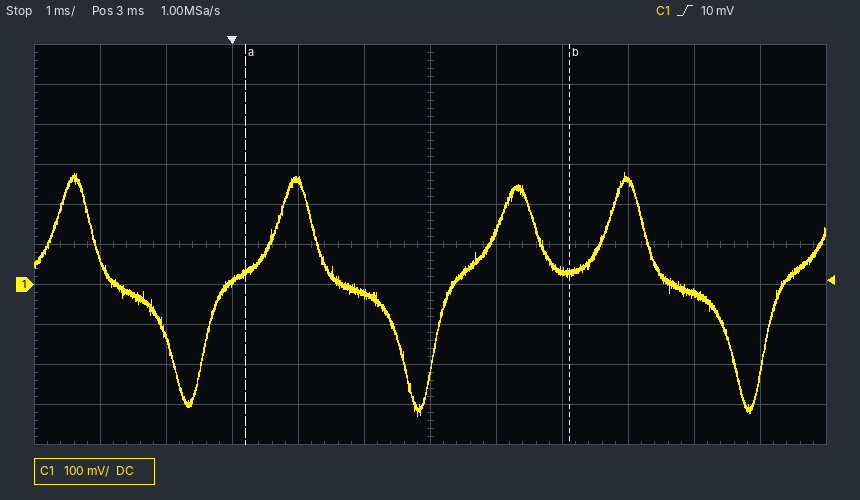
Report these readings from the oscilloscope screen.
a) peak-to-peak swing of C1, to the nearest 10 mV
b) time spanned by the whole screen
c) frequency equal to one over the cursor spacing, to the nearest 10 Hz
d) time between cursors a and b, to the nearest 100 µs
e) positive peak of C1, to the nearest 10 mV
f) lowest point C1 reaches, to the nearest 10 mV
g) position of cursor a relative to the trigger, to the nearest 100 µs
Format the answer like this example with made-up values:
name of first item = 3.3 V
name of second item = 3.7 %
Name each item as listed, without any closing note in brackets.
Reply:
peak-to-peak swing of C1, to the nearest 10 mV = 610 mV
time spanned by the whole screen = 12 ms
frequency equal to one over the cursor spacing, to the nearest 10 Hz = 200 Hz
time between cursors a and b, to the nearest 100 µs = 4.9 ms
positive peak of C1, to the nearest 10 mV = 280 mV
lowest point C1 reaches, to the nearest 10 mV = -330 mV
position of cursor a relative to the trigger, to the nearest 100 µs = +200 µs
